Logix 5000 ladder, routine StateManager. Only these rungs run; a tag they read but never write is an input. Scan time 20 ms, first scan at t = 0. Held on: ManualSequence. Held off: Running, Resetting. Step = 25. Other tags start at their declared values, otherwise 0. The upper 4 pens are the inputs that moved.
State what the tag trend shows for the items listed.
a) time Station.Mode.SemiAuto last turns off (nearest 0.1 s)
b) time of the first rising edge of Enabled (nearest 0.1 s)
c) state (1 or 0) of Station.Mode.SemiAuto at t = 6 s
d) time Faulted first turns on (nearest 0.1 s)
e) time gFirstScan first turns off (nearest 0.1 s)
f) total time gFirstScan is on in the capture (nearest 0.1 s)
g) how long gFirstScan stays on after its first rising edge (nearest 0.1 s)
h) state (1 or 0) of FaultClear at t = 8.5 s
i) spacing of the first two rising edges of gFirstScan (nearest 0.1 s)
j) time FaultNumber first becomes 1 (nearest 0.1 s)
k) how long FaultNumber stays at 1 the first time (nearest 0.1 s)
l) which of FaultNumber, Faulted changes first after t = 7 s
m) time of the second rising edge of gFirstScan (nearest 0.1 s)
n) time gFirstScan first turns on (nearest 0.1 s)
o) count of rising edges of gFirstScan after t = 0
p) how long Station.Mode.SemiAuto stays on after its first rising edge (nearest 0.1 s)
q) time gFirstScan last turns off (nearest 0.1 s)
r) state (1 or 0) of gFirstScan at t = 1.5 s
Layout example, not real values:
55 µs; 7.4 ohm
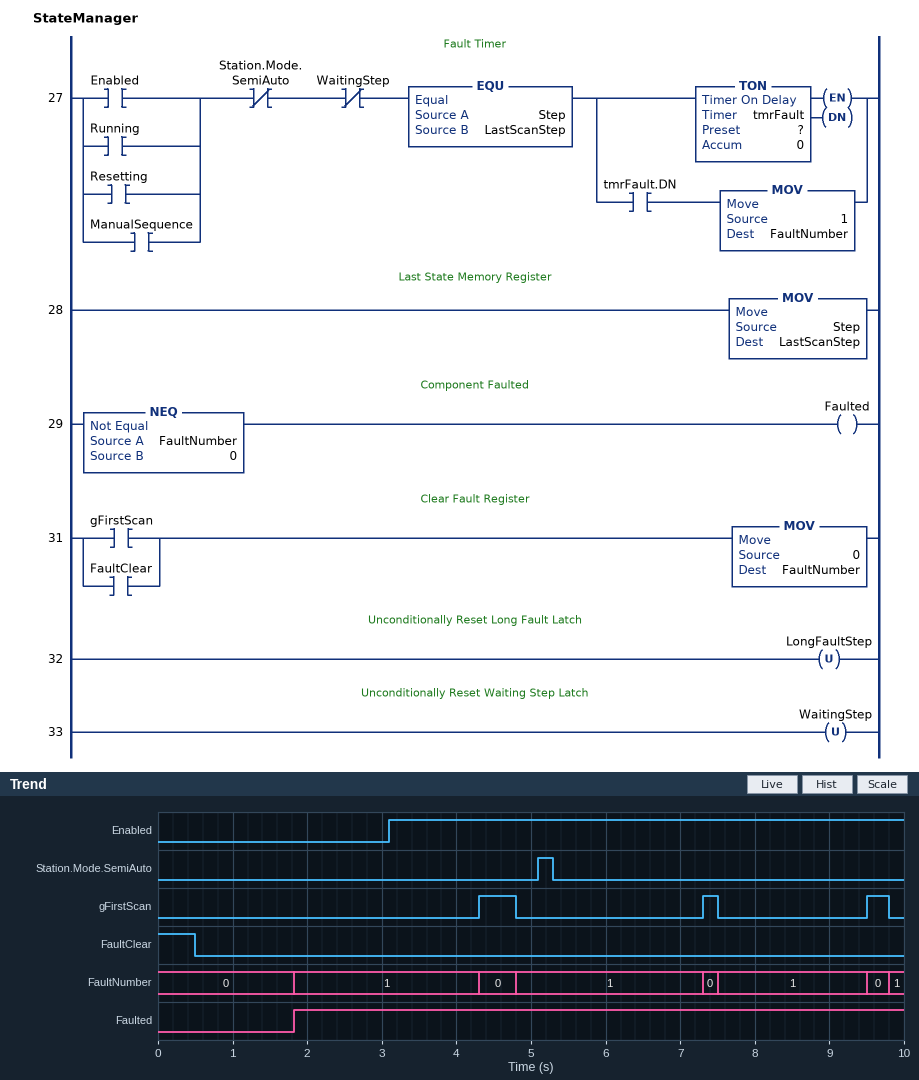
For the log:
5.3 s; 3.1 s; 0; 1.8 s; 4.8 s; 1.0 s; 0.5 s; 0; 3.0 s; 1.8 s; 2.5 s; FaultNumber; 7.3 s; 4.3 s; 3; 0.2 s; 9.8 s; 0
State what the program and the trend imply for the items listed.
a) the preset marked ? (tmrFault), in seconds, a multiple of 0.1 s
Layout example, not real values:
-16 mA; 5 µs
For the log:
1.8 s
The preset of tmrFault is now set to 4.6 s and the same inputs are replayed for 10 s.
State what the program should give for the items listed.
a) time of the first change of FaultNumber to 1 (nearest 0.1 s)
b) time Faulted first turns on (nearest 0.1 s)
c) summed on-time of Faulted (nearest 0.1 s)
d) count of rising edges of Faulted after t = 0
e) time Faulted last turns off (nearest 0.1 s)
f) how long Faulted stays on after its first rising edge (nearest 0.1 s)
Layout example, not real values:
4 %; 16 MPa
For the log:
4.8 s; 4.6 s; 2.8 s; 2; 7.3 s; 2.7 s
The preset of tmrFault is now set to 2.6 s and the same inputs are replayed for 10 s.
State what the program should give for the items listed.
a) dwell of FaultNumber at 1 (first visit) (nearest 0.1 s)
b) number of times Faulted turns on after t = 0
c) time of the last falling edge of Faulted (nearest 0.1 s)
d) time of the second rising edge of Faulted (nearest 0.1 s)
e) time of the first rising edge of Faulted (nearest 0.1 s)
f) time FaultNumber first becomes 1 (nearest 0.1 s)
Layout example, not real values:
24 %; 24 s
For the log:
1.7 s; 2; 7.3 s; 7.9 s; 2.6 s; 2.6 s
